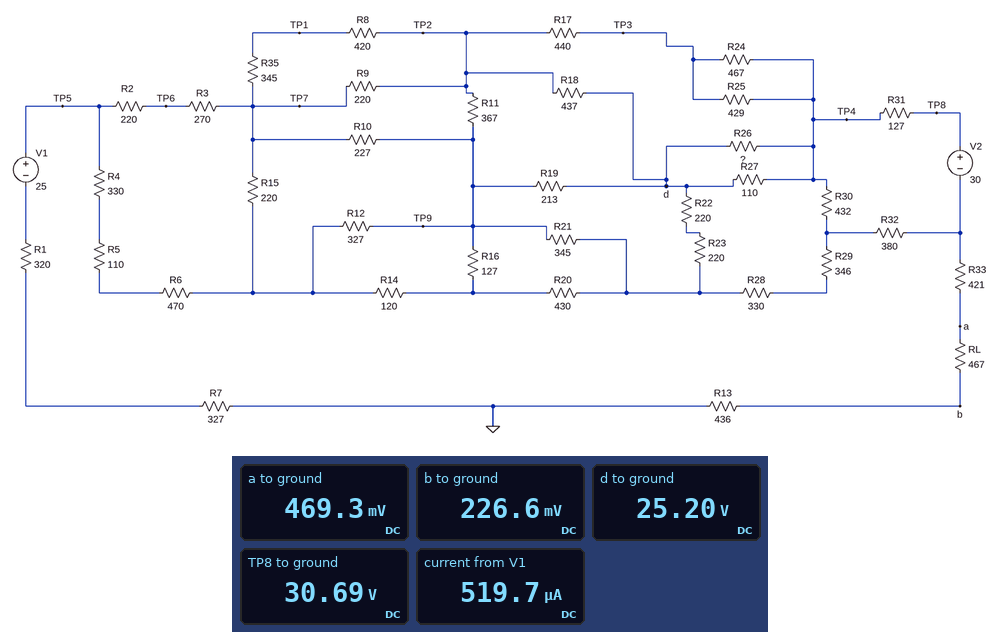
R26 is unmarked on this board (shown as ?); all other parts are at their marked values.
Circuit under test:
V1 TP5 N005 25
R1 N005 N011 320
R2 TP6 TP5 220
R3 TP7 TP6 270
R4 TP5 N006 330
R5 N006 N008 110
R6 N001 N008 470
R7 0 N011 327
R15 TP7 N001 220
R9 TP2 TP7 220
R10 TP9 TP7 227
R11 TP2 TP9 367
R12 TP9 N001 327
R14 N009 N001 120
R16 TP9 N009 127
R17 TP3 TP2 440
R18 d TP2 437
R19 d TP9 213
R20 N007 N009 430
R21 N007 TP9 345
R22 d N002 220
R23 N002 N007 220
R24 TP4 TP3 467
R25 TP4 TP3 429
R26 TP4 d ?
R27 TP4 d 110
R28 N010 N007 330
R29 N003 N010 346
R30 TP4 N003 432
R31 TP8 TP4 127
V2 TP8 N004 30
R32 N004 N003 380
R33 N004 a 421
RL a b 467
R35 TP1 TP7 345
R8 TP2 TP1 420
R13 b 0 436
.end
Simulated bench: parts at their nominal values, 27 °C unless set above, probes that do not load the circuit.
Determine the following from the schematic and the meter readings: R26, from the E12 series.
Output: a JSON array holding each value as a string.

["330 Ω"]
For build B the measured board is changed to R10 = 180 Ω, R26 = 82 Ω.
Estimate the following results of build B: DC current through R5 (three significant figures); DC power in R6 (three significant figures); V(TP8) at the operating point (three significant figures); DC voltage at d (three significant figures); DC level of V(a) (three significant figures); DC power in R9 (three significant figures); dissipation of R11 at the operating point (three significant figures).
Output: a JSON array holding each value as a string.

["284 µA", "37.8 µW", "30.6 V", "25.4 V", "390 mV", "283 µW", "409 µW"]
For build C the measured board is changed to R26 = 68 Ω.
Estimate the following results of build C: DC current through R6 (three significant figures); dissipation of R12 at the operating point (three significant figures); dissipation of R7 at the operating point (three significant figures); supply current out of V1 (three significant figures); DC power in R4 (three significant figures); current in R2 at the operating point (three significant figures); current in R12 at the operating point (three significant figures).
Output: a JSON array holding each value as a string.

["283 µA", "5.61 µW", "56.3 µW", "415 µA", "26.5 µW", "132 µA", "131 µA"]
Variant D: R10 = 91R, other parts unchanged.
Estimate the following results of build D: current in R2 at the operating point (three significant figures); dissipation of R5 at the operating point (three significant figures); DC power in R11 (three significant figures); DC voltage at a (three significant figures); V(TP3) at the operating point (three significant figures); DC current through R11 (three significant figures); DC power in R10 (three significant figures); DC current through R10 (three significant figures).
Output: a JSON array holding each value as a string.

["232 µA", "10.1 µW", "407 µW", "483 mV", "25.6 V", "1.05 mA", "120 µW", "1.15 mA"]
